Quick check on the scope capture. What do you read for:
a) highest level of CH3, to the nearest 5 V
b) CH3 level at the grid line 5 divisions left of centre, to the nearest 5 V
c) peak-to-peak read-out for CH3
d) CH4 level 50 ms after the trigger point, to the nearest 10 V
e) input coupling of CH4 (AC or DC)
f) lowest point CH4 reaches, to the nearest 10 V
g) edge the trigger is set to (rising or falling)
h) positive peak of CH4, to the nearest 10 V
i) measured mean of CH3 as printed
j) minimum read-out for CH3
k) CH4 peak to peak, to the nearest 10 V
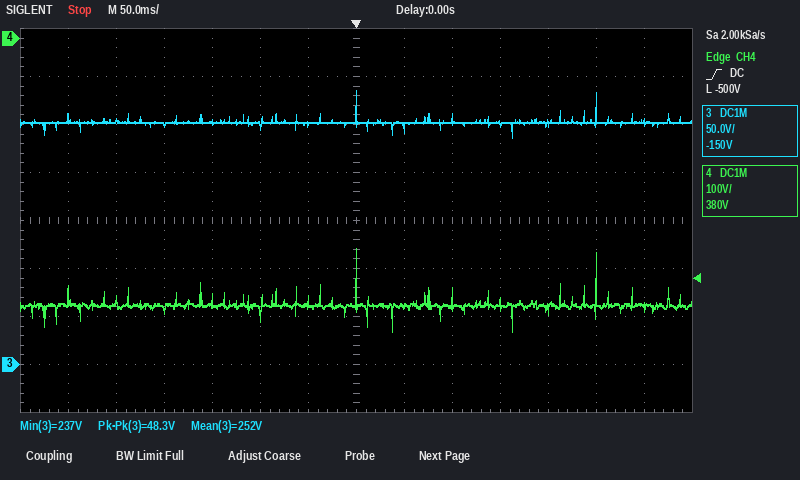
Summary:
285 V
255 V
48.3 V
-560 V
DC
-610 V
rising
-440 V
252 V
237 V
170 V
